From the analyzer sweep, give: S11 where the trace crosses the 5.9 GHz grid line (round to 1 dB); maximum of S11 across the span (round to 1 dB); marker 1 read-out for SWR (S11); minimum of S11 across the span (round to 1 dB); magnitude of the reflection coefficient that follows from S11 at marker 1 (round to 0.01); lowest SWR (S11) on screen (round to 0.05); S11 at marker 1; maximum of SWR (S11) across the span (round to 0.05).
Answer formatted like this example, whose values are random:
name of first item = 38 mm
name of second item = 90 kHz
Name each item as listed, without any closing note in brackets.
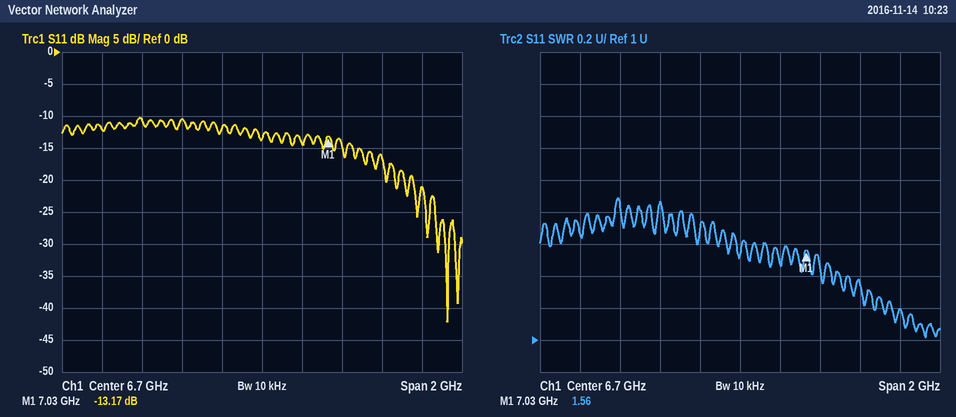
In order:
S11 where the trace crosses the 5.9 GHz grid line = -12 dB
maximum of S11 across the span = -10 dB
marker 1 read-out for SWR = 1.56
minimum of S11 across the span = -42 dB
magnitude of the reflection coefficient that follows from S11 at marker 1 = 0.22
lowest SWR (S11) on screen = 1.00
S11 at marker 1 = -13.17 dB
maximum of SWR (S11) across the span = 1.90
